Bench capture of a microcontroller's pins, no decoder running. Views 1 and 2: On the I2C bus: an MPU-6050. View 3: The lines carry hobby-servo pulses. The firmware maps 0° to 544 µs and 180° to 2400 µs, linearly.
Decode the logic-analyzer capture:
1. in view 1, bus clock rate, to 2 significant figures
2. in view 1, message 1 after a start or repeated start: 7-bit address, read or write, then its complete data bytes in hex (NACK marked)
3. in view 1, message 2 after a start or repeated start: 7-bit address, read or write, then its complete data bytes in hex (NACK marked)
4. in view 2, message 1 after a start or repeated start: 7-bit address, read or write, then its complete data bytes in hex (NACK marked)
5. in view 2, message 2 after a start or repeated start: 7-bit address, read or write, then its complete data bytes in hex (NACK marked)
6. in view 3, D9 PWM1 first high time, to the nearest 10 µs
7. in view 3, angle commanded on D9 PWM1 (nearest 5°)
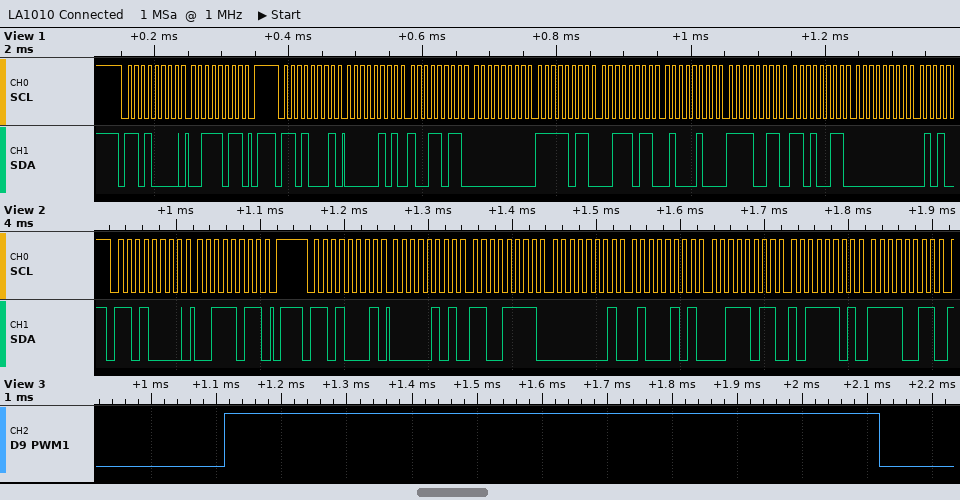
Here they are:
100 kHz
0x68 write: 3B
0x68 read: 05 9B 00 FB 3B 44 F3 D3 00
0x68 write: 3B
0x68 read: 05 CF 01 45 3B BD F3
1010 µs
45°
